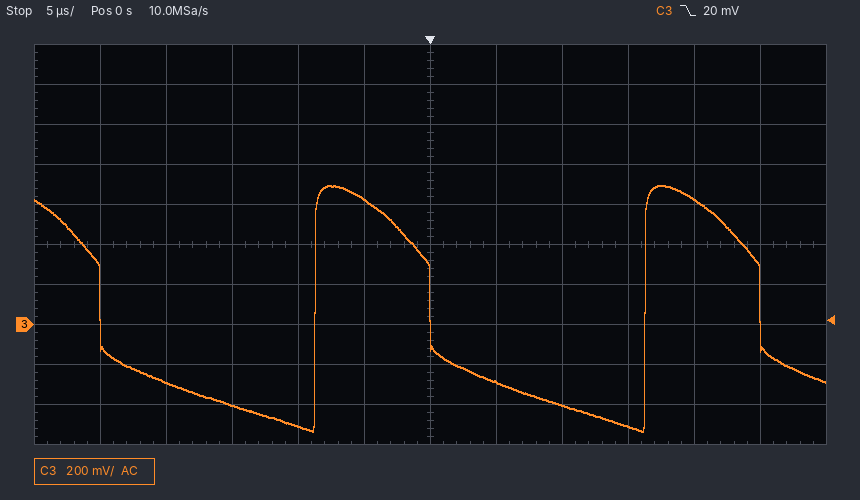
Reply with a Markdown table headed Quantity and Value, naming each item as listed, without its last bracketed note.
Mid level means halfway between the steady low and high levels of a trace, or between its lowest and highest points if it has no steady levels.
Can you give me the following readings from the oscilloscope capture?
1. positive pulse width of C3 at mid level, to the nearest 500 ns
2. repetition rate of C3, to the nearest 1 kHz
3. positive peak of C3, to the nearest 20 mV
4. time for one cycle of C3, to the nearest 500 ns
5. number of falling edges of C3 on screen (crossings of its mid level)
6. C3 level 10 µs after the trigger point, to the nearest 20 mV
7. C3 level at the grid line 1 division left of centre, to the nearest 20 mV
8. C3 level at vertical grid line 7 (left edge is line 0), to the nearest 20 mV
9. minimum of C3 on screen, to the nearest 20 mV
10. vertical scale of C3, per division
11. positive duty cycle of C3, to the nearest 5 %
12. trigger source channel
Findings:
| Quantity | Value |
|---|---|
| positive pulse width of C3 at mid level, to the nearest 500 ns | 8.5 µs |
| repetition rate of C3, to the nearest 1 kHz | 40 kHz |
| positive peak of C3, to the nearest 20 mV | 700 mV |
| time for one cycle of C3, to the nearest 500 ns | 25.0 µs |
| number of falling edges of C3 on screen | 3 |
| C3 level 10 µs after the trigger point, to the nearest 20 mV | -400 mV |
| C3 level at the grid line 1 division left of centre, to the nearest 20 mV | 620 mV |
| C3 level at vertical grid line 7 (left edge is line 0), to the nearest 20 mV | -280 mV |
| minimum of C3 on screen, to the nearest 20 mV | -540 mV |
| vertical scale of C3, per division | 200 mV |
| positive duty cycle of C3, to the nearest 5 % | 35 % |
| trigger source channel | C3 |
